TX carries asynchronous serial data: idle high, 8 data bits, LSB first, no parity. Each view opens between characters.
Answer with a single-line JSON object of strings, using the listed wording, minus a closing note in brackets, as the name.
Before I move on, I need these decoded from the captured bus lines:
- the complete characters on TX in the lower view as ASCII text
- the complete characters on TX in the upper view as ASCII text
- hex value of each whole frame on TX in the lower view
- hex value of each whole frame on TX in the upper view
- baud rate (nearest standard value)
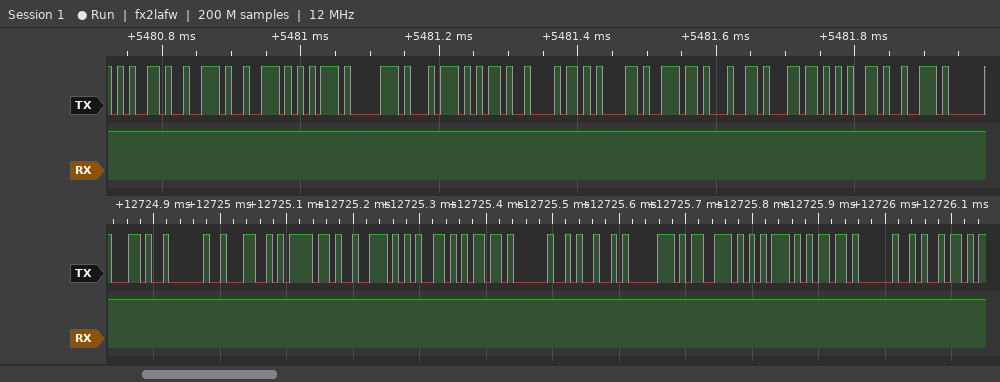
{"the complete characters on TX in the lower view as ASCII text": "\", Lorem Ipsum i\"", "the complete characters on TX in the upper view as ASCII text": "\"errupt-handler\"", "hex value of each whole frame on TX in the lower view": "2C, 20, 4C, 6F, 72, 65, 6D, 20, 49, 70, 73, 75, 6D, 20, 69", "hex value of each whole frame on TX in the upper view": "65, 72, 72, 75, 70, 74, 2D, 68, 61, 6E, 64, 6C, 65, 72", "baud rate": "115200 baud"}
